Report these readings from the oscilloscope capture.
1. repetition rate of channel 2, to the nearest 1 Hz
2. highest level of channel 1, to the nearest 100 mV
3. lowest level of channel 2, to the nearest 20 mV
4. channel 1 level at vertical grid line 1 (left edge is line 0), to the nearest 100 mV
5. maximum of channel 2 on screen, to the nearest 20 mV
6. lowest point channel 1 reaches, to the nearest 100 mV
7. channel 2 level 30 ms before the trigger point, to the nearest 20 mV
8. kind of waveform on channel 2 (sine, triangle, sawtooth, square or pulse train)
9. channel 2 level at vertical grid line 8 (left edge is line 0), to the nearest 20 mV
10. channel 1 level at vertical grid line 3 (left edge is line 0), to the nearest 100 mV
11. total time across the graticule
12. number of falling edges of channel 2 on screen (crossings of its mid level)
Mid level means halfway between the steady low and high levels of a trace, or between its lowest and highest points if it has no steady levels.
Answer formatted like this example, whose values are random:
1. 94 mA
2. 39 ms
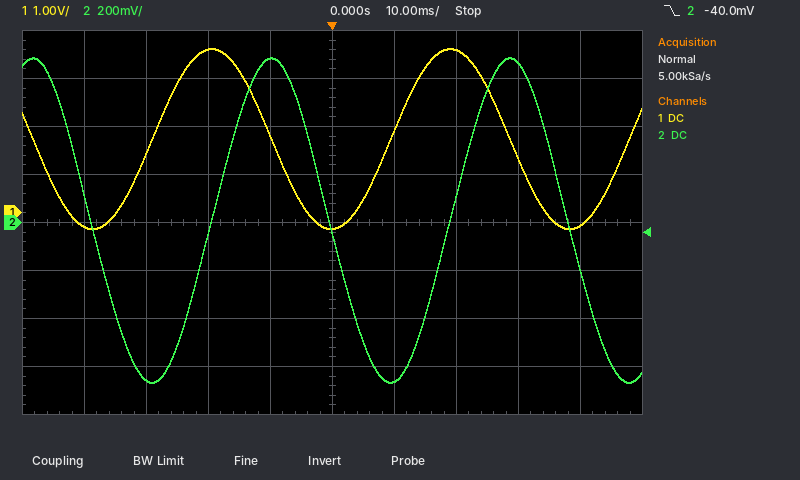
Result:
1. 26 Hz
2. 3.4 V
3. -660 mV
4. -300 mV
5. 680 mV
6. -300 mV
7. -660 mV
8. sine
9. 660 mV
10. 3.4 V
11. 100 ms
12. 3
